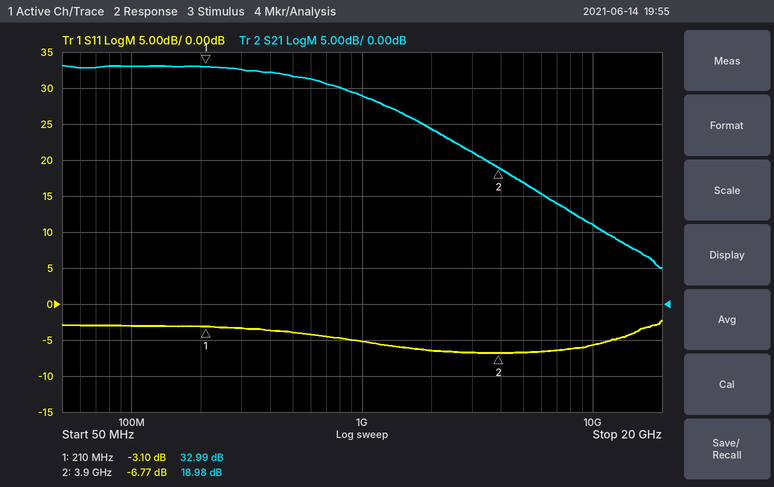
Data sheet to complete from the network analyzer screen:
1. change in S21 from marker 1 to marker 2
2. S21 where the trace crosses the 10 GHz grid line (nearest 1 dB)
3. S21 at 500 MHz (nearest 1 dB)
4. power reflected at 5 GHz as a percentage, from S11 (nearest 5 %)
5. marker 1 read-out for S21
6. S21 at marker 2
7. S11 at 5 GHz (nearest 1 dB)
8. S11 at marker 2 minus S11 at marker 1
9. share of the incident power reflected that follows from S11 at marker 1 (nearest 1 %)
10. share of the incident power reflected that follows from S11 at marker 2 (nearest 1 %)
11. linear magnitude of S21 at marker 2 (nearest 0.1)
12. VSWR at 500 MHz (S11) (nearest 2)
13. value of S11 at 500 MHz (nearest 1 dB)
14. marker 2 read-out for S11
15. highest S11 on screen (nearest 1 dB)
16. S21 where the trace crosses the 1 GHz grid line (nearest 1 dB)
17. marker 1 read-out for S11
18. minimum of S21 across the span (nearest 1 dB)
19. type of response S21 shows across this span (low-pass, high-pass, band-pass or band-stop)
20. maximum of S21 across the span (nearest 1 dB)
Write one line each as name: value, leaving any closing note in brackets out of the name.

change in S21 from marker 1 to marker 2: -14.01 dB
S21 where the trace crosses the 10 GHz grid line: 11 dB
S21 at 500 MHz: 32 dB
power reflected at 5 GHz as a percentage, from S11: 20 %
marker 1 read-out for S21: 32.99 dB
S21 at marker 2: 18.98 dB
S11 at 5 GHz: -7 dB
S11 at marker 2 minus S11 at marker 1: -3.67 dB
share of the incident power reflected that follows from S11 at marker 1: 49 %
share of the incident power reflected that follows from S11 at marker 2: 21 %
linear magnitude of S21 at marker 2: 8.9
VSWR at 500 MHz (S11): 4
value of S11 at 500 MHz: -4 dB
marker 2 read-out for S11: -6.77 dB
highest S11 on screen: -2 dB
S21 where the trace crosses the 1 GHz grid line: 29 dB
marker 1 read-out for S11: -3.10 dB
minimum of S21 across the span: 5 dB
type of response S21 shows across this span: low-pass
maximum of S21 across the span: 33 dB
